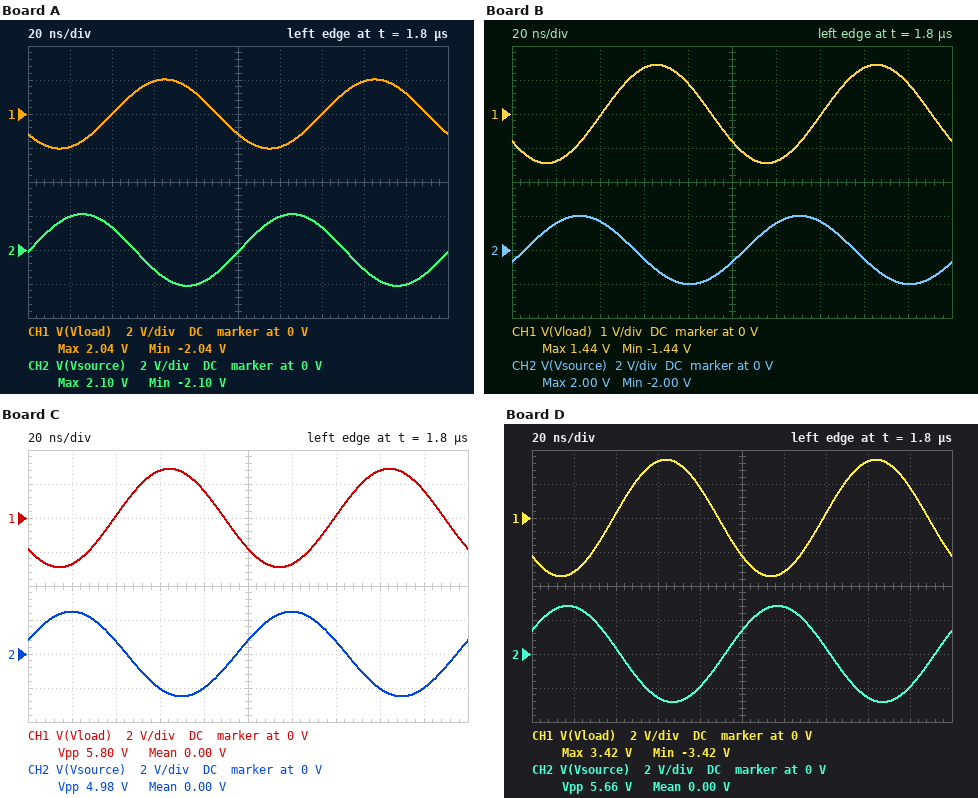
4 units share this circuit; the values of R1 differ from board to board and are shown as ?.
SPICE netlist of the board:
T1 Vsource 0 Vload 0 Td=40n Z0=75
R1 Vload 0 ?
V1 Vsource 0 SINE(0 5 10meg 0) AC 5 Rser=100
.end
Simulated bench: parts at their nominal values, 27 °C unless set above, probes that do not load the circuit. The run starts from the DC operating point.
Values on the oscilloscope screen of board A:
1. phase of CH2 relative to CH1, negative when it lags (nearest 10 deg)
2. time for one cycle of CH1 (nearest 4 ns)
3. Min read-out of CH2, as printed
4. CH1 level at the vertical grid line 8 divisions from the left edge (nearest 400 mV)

140 deg
100 ns
-2.10 V
2.0 V
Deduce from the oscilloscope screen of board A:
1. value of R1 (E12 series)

68 Ω
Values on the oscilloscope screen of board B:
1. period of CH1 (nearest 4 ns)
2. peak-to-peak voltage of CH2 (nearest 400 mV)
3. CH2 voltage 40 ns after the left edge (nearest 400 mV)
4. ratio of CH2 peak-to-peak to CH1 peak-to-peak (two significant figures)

100 ns
4.0 V
1.6 V
1.4
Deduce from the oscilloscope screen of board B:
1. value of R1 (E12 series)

39 Ω
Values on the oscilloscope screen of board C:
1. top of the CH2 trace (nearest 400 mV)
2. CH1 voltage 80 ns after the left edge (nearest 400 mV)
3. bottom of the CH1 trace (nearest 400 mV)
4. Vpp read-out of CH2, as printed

2.4 V
1.6 V
-2.8 V
4.98 V
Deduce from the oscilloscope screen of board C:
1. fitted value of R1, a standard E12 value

150 Ω
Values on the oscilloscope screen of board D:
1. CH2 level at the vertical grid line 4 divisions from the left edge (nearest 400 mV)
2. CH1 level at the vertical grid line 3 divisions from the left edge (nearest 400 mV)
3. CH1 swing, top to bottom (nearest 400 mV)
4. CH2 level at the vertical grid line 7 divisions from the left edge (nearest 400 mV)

-2.0 V
3.2 V
6.8 V
400 mV
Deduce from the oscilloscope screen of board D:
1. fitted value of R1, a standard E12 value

270 Ω
